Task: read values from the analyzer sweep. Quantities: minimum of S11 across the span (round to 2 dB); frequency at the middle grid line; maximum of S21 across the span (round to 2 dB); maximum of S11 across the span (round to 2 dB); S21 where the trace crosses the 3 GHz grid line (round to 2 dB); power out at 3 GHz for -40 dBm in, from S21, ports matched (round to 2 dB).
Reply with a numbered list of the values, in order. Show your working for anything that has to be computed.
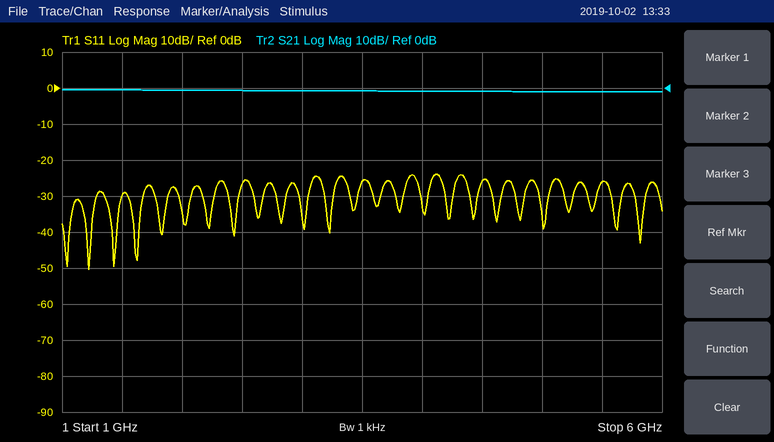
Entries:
1. -50 dB
2. 3.5 GHz
3. 0 dB
4. -24 dB
5. 0 dB
6. -40 dBm + (0 dB) = -40 dBm
